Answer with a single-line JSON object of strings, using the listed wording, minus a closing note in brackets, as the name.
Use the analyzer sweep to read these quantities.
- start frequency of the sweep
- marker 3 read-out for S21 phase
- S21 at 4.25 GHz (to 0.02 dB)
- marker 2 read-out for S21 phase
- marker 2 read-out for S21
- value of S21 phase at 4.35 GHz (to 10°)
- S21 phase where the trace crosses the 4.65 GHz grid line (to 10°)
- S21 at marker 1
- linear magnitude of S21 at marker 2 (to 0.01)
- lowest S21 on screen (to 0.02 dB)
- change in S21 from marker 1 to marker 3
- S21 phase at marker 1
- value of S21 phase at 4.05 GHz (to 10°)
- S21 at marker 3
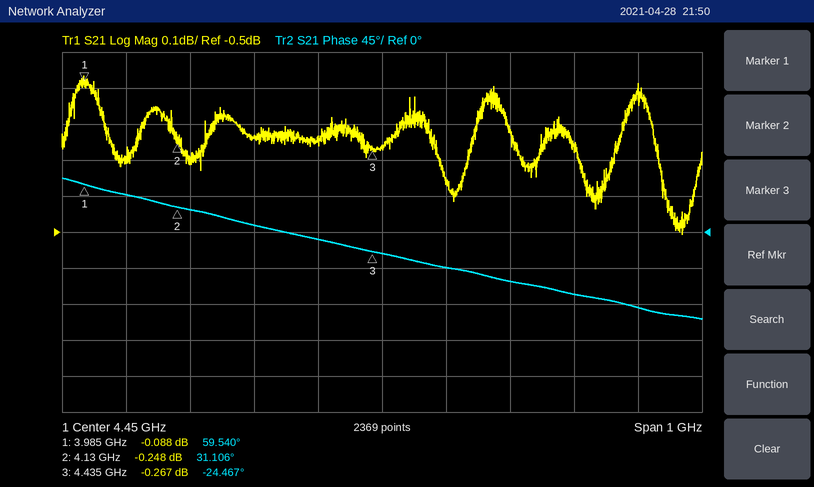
{"start frequency of the sweep": "3.95 GHz", "marker 3 read-out for S21 phase": "-24.467°", "S21 at 4.25 GHz": "-0.24 dB", "marker 2 read-out for S21 phase": "31.106°", "marker 2 read-out for S21": "-0.248 dB", "value of S21 phase at 4.35 GHz": "-10°", "S21 phase where the trace crosses the 4.65 GHz grid line": "-60°", "S21 at marker 1": "-0.088 dB", "linear magnitude of S21 at marker 2": "0.97", "lowest S21 on screen": "-0.50 dB", "change in S21 from marker 1 to marker 3": "-0.179 dB", "S21 phase at marker 1": "59.540°", "value of S21 phase at 4.05 GHz": "50°", "S21 at marker 3": "-0.267 dB"}
